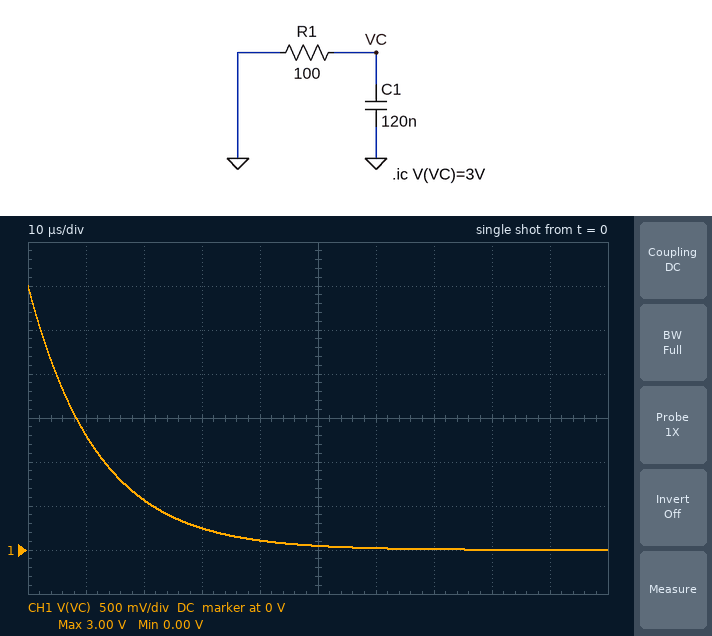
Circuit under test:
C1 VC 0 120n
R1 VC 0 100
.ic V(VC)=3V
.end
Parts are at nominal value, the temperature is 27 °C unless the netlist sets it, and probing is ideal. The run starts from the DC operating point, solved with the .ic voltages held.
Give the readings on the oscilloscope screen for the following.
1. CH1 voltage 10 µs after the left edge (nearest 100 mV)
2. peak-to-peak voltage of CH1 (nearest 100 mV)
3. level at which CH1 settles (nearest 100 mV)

1.3 V
3.0 V
0 V
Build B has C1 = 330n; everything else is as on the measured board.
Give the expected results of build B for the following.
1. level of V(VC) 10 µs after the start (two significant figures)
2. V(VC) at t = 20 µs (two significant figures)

2.2 V
1.6 V
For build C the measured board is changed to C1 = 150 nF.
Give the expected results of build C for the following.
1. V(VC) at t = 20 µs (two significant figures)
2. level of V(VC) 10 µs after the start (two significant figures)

790 mV
1.5 V
